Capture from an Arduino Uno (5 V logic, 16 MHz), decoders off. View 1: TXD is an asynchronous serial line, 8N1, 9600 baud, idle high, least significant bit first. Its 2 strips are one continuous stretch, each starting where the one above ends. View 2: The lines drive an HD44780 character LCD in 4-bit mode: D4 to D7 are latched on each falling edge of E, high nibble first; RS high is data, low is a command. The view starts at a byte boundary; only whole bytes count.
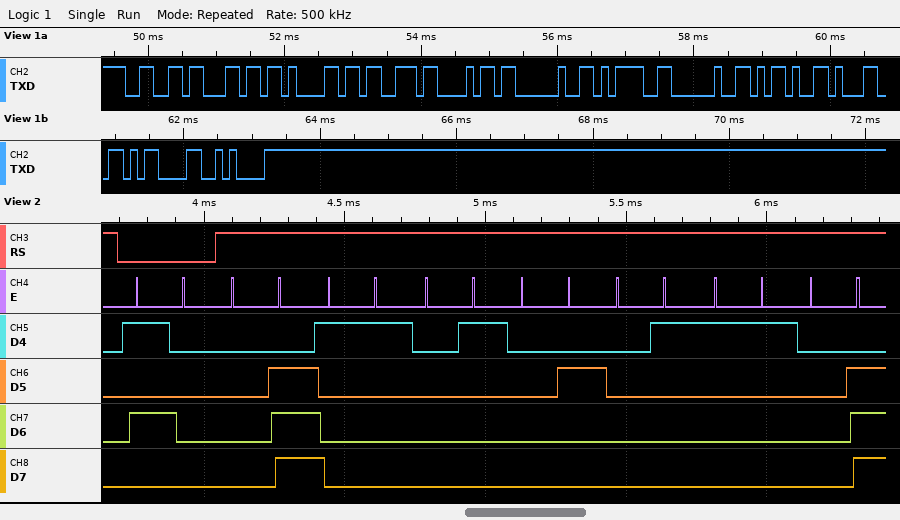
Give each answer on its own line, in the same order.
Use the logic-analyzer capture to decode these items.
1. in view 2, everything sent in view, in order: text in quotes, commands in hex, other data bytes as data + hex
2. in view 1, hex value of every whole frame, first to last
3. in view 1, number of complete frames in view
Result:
0x50 data 0E 11 01 02 01 11 0E
66 6C 61 73 68 20 3D 20 2D 31 0D 0A
12
